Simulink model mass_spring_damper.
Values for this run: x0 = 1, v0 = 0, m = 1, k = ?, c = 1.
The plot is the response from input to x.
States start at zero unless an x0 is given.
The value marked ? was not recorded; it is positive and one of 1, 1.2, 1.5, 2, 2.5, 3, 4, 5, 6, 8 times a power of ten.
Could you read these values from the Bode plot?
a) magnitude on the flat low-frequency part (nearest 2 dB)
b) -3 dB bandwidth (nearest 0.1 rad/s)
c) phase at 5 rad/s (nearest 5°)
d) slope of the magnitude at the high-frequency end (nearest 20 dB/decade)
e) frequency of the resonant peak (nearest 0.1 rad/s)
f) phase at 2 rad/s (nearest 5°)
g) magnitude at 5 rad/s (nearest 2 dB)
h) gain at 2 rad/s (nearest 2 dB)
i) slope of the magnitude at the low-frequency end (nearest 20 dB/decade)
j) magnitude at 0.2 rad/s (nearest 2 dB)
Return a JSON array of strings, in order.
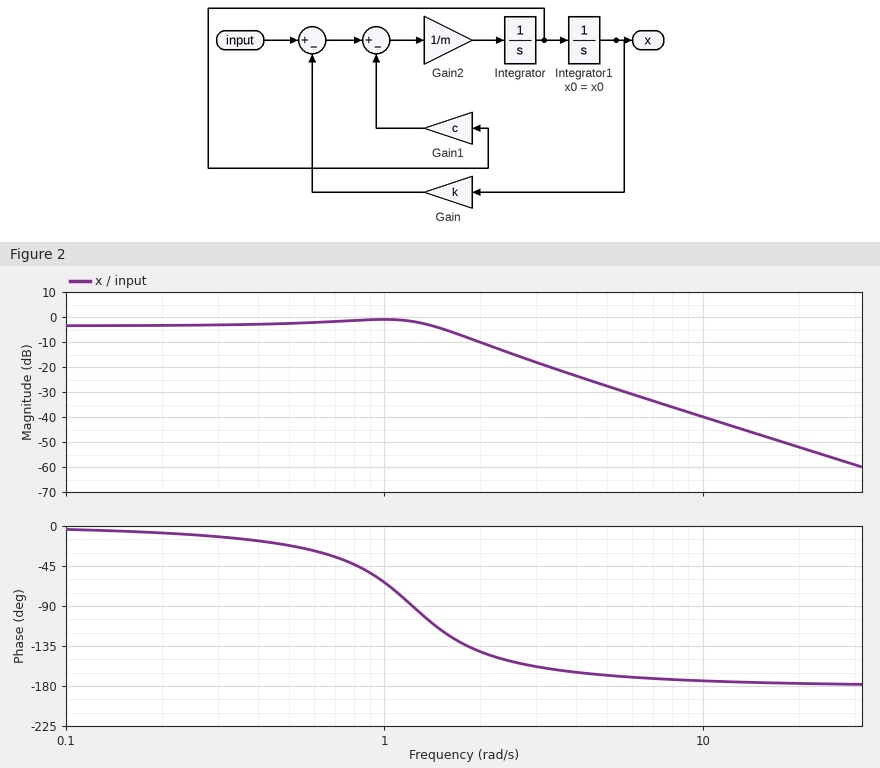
["-4 dB", "1.7 rad/s", "-170°", "-40 dB/decade", "1.0 rad/s", "-140°", "-28 dB", "-10 dB", "0 dB/decade", "-4 dB"]
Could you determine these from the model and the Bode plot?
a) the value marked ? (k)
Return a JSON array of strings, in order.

["1.5"]
